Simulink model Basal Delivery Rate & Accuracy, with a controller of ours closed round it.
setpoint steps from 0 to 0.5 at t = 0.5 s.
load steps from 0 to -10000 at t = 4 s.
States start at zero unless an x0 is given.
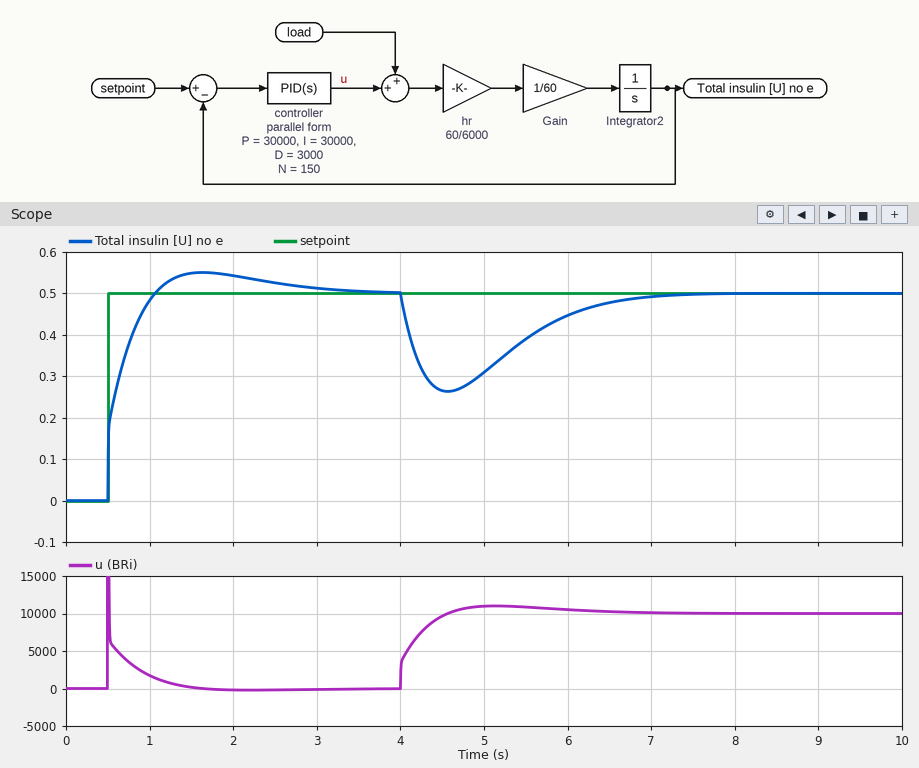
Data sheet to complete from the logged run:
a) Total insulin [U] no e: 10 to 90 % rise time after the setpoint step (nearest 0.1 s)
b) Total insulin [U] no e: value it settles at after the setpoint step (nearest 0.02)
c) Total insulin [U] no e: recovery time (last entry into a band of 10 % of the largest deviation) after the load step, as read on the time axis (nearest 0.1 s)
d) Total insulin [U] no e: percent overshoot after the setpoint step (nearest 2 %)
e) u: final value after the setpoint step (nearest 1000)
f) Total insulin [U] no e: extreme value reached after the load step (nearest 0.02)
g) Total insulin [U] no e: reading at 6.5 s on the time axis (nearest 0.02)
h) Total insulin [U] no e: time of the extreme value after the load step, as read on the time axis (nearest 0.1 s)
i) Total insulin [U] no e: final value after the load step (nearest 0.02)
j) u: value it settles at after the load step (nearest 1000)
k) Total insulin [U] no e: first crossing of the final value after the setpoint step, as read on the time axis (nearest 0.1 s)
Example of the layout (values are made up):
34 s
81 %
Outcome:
0.4 s
0.50
6.5 s
10 %
0
0.26
0.48
4.6 s
0.50
10000
1.1 s
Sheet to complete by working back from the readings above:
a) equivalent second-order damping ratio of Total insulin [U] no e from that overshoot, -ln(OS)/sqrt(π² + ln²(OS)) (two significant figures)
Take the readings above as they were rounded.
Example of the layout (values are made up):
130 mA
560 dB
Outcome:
0.59
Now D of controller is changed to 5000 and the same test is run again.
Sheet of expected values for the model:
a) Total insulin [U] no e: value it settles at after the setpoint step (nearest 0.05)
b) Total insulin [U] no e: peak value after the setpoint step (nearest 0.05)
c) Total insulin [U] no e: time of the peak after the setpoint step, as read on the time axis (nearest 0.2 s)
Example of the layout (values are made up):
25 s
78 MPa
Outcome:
0.50
0.55
1.8 s
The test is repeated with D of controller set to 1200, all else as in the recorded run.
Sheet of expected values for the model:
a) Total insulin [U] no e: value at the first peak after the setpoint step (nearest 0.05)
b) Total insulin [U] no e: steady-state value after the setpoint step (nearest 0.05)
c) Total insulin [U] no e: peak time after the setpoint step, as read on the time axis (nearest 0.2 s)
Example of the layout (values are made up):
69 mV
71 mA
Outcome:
0.55
0.50
1.4 s
